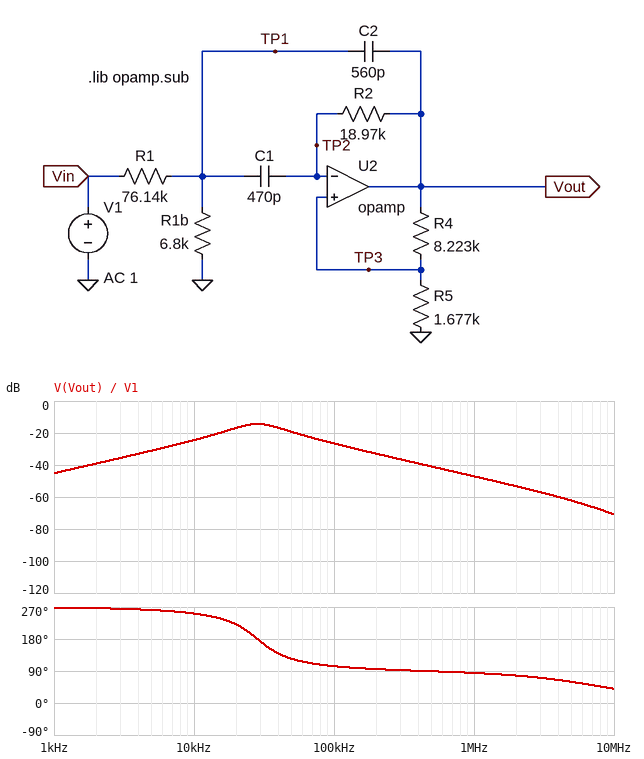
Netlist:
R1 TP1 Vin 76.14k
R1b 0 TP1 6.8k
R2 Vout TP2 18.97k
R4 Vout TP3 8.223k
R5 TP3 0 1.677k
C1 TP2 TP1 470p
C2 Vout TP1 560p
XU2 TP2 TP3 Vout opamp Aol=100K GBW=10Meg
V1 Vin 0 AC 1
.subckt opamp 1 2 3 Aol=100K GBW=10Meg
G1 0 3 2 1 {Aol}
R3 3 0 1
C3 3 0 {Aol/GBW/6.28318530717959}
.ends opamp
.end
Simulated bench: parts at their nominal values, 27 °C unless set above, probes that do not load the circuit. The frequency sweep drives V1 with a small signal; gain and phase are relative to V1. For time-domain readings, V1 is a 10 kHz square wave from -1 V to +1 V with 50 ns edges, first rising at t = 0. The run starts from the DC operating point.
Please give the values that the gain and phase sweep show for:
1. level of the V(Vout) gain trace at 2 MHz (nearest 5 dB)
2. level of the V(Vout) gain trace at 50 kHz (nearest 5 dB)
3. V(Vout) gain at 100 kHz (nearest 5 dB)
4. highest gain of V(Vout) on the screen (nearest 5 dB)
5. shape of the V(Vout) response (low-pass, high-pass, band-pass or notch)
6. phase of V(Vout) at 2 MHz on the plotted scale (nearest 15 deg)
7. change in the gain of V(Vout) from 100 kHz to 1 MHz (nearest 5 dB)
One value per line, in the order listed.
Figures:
-55 dB
-20 dB
-25 dB
-15 dB
band-pass
75 deg
-20 dB
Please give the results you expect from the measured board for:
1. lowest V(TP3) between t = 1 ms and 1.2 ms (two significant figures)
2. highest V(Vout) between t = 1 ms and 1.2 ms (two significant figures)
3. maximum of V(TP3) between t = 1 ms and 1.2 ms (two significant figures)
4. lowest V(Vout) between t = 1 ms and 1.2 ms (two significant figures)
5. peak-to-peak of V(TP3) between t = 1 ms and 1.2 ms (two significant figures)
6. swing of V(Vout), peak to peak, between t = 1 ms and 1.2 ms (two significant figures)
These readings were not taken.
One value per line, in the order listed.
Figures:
-32 mV
190 mV
32 mV
-190 mV
63 mV
370 mV
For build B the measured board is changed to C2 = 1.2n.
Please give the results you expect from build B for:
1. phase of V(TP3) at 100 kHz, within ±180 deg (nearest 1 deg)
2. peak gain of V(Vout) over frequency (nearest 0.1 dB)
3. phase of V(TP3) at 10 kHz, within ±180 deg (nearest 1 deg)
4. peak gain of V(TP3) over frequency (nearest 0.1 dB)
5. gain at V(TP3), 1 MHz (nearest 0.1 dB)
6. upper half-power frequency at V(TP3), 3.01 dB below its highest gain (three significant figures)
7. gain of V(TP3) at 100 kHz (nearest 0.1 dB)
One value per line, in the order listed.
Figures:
101 deg
-19.8 dB
-126 deg
-35.2 dB
-69.1 dB
32.2 kHz
-48.9 dB
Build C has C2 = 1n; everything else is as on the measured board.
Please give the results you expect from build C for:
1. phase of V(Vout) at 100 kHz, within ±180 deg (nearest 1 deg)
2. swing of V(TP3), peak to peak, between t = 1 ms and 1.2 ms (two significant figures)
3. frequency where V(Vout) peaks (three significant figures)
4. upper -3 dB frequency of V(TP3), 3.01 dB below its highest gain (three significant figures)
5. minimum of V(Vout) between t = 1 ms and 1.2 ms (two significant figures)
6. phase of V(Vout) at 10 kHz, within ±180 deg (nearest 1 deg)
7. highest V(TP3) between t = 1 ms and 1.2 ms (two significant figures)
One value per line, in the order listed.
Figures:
102 deg
43 mV
21.3 kHz
34.2 kHz
-130 mV
-121 deg
21 mV
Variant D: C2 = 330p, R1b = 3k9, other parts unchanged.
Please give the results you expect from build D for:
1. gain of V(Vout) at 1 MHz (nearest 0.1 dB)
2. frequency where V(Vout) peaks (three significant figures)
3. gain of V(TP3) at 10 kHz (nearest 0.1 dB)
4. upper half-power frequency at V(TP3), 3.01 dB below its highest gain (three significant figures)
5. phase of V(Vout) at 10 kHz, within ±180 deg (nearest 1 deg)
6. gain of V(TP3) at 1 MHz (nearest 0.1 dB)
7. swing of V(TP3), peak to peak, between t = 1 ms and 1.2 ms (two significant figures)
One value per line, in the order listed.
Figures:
-42.6 dB
47.7 kHz
-44.7 dB
56.7 kHz
-94 deg
-58.0 dB
86 mV
